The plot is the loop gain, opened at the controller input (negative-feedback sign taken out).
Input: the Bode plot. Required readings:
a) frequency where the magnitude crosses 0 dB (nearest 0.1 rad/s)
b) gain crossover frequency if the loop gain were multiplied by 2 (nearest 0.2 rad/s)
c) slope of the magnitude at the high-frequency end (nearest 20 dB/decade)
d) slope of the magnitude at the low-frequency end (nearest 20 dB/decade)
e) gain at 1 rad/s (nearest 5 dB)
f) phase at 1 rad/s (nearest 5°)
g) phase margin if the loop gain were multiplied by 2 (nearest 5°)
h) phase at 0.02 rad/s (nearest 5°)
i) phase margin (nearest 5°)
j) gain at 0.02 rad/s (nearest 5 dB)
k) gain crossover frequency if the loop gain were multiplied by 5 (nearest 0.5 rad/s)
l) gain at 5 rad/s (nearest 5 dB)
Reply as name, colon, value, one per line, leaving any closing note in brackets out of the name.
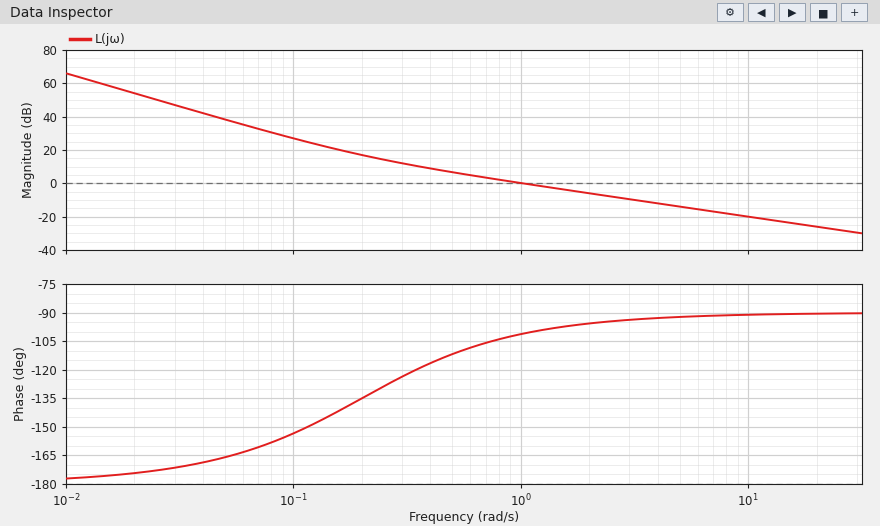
frequency where the magnitude crosses 0 dB: 1.0 rad/s
gain crossover frequency if the loop gain were multiplied by 2: 2.0 rad/s
slope of the magnitude at the high-frequency end: -20 dB/decade
slope of the magnitude at the low-frequency end: -40 dB/decade
gain at 1 rad/s: 0 dB
phase at 1 rad/s: -100°
phase margin if the loop gain were multiplied by 2: 85°
phase at 0.02 rad/s: -175°
phase margin: 80°
gain at 0.02 rad/s: 55 dB
gain crossover frequency if the loop gain were multiplied by 5: 5.0 rad/s
gain at 5 rad/s: -15 dB
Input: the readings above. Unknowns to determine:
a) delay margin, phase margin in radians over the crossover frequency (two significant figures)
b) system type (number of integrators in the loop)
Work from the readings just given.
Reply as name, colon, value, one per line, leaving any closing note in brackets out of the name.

delay margin, phase margin in radians over the crossover frequency: 1.4 s
system type: 2
